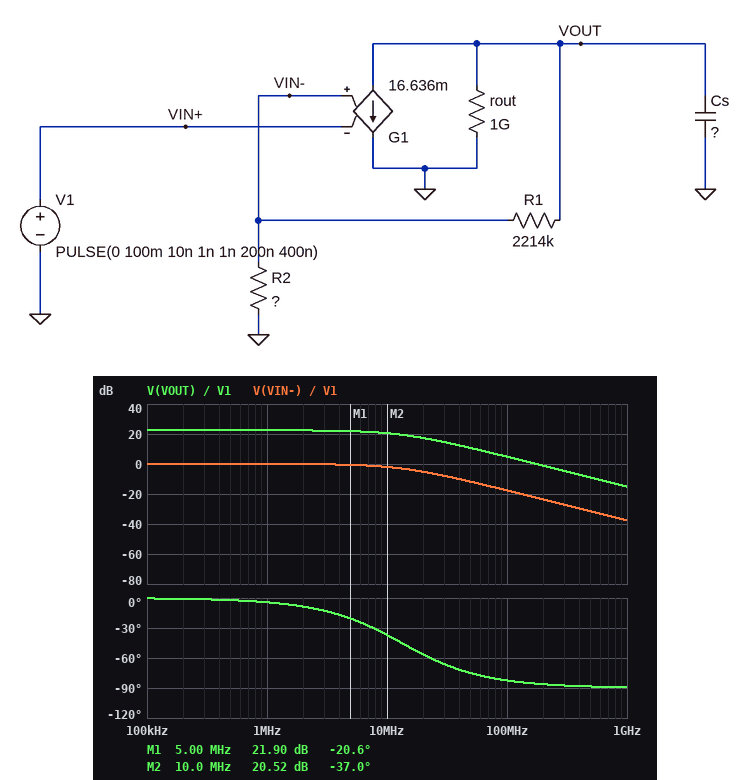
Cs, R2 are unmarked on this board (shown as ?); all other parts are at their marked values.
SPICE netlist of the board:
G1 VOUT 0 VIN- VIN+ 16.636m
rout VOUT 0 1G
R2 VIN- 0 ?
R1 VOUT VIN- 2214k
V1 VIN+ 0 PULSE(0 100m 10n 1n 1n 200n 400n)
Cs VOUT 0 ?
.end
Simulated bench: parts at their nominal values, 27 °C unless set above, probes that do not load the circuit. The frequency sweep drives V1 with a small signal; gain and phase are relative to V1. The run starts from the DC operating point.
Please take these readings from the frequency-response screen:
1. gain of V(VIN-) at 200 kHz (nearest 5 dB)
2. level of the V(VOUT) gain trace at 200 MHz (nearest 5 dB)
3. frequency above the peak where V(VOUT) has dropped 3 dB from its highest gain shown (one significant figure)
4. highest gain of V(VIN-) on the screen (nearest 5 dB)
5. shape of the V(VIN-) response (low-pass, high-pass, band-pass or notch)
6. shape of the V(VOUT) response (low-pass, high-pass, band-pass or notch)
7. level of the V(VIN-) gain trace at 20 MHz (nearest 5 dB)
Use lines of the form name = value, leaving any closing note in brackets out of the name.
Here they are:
gain of V(VIN-) at 200 kHz = 0 dB
level of the V(VOUT) gain trace at 200 MHz = 0 dB
frequency above the peak where V(VOUT) has dropped 3 dB from its highest gain shown = 10 MHz
highest gain of V(VIN-) on the screen = 0 dB
shape of the V(VIN-) response = low-pass
shape of the V(VOUT) response = low-pass
level of the V(VIN-) gain trace at 20 MHz = -5 dB
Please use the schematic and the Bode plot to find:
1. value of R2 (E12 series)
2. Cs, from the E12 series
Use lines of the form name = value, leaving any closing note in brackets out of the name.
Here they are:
value of R2 = 180 kΩ
Cs, from the E12 series = 15 pF
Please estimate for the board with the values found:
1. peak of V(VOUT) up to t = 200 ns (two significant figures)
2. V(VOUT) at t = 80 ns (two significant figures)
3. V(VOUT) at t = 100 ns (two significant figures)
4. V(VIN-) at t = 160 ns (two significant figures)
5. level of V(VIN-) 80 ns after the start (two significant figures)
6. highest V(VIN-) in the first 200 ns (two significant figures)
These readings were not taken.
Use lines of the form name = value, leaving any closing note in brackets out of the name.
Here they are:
peak of V(VOUT) up to t = 200 ns = 1.3 V
V(VOUT) at t = 80 ns = 1.3 V
V(VOUT) at t = 100 ns = 1.3 V
V(VIN-) at t = 160 ns = 100 mV
level of V(VIN-) 80 ns after the start = 100 mV
highest V(VIN-) in the first 200 ns = 100 mV
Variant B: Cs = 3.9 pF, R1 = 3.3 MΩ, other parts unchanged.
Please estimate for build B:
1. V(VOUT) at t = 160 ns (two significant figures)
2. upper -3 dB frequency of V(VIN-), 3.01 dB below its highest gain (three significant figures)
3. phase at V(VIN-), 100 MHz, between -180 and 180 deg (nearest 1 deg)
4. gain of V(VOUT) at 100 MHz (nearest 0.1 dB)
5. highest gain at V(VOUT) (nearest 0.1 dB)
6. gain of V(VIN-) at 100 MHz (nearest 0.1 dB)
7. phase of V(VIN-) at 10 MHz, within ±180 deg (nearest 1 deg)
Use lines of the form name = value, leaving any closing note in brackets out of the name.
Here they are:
V(VOUT) at t = 160 ns = 1.9 V
upper -3 dB frequency of V(VIN-), 3.01 dB below its highest gain = 35.1 MHz
phase at V(VIN-), 100 MHz, between -180 and 180 deg = -71 deg
gain of V(VOUT) at 100 MHz = 16.1 dB
highest gain at V(VOUT) = 25.7 dB
gain of V(VIN-) at 100 MHz = -9.6 dB
phase of V(VIN-) at 10 MHz, within ±180 deg = -16 deg
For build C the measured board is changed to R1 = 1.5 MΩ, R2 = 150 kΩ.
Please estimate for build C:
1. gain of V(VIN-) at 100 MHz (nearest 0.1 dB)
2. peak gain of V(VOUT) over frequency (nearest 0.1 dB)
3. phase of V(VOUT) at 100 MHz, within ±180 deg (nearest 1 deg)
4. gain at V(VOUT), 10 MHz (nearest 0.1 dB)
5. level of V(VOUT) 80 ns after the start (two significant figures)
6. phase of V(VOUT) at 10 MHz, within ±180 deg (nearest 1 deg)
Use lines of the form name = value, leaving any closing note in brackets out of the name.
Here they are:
gain of V(VIN-) at 100 MHz = -16.0 dB
peak gain of V(VOUT) over frequency = 20.8 dB
phase of V(VOUT) at 100 MHz, within ±180 deg = -81 deg
gain at V(VOUT), 10 MHz = 19.4 dB
level of V(VOUT) 80 ns after the start = 1.1 V
phase of V(VOUT) at 10 MHz, within ±180 deg = -32 deg
